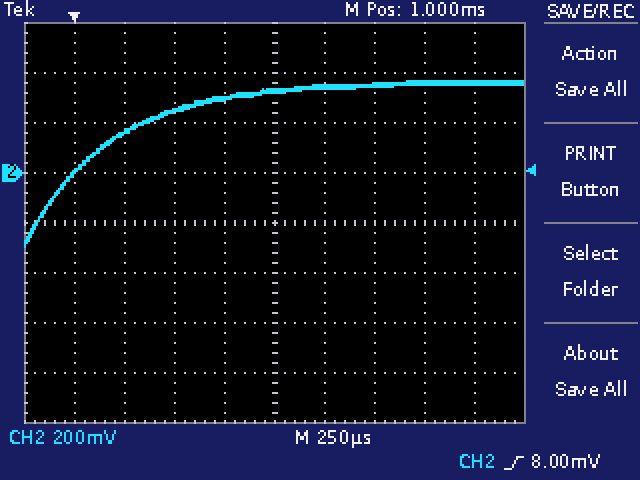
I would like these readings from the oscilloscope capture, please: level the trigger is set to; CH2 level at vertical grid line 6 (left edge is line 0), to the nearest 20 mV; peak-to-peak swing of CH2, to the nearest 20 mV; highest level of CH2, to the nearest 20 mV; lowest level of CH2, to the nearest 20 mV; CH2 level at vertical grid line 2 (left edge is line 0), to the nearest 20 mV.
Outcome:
8.00 mV
340 mV
660 mV
360 mV
-300 mV
160 mV
